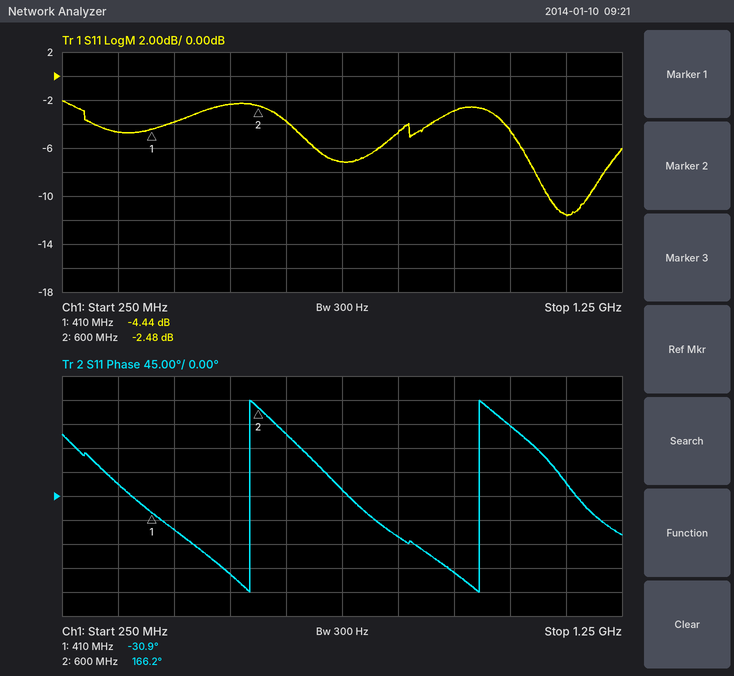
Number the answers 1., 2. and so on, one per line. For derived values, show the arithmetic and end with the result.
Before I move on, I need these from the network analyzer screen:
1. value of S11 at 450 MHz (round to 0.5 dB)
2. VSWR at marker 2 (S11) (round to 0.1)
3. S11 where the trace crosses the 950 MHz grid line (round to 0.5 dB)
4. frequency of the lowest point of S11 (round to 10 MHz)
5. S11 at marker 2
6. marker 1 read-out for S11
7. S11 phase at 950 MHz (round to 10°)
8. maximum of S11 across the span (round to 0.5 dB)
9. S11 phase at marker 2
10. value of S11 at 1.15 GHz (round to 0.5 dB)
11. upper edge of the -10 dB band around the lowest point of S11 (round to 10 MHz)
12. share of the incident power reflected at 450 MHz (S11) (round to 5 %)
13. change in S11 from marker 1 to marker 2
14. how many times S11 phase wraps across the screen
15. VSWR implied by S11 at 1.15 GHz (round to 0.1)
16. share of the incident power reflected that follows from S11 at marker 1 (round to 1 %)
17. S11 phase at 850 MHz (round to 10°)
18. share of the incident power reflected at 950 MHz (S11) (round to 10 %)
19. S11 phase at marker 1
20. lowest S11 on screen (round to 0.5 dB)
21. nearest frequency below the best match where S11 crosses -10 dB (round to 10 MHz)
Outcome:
1. -4.0 dB
2. (1 + 0.7516)/(1 − 0.7516) ≈ 7.1
3. -3.0 dB
4. 1.15 GHz
5. -2.48 dB
6. -4.44 dB
7. -140°
8. -2.0 dB
9. 166.2°
10. -11.5 dB
11. 1.19 GHz
12. 10^(-4/10) ≈ 40 %
13. -2.48 − (-4.44) = 1.96 dB
14. 2
15. |Γ| = 10^(-11.5/20) = 0.2661; VSWR = (1 + 0.2661)/(1 − 0.2661) ≈ 1.7
16. 10^(-4.44/10) ≈ 36 %
17. -80°
18. 10^(-3/10) ≈ 50 %
19. -30.9°
20. -11.5 dB
21. 1.12 GHz
